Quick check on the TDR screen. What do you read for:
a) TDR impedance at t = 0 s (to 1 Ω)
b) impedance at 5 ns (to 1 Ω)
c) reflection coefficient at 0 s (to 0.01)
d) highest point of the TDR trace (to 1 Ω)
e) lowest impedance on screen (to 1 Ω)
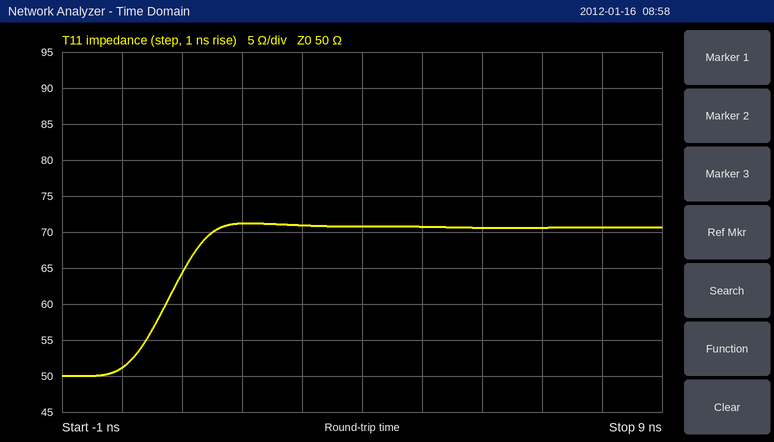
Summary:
51 Ω
71 Ω
+0.01
71 Ω
50 Ω
